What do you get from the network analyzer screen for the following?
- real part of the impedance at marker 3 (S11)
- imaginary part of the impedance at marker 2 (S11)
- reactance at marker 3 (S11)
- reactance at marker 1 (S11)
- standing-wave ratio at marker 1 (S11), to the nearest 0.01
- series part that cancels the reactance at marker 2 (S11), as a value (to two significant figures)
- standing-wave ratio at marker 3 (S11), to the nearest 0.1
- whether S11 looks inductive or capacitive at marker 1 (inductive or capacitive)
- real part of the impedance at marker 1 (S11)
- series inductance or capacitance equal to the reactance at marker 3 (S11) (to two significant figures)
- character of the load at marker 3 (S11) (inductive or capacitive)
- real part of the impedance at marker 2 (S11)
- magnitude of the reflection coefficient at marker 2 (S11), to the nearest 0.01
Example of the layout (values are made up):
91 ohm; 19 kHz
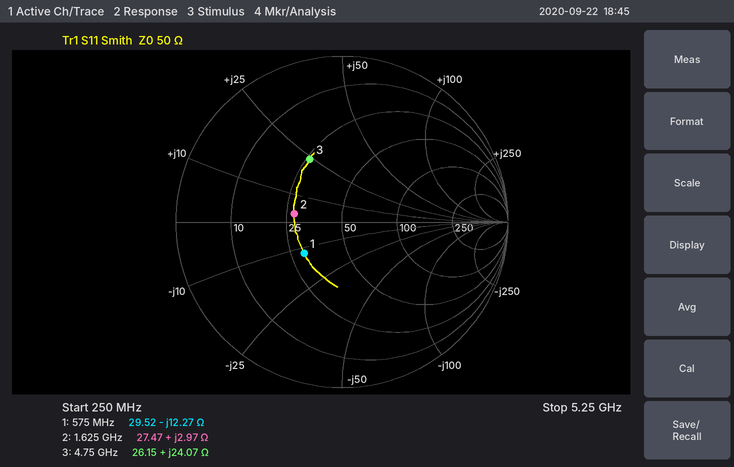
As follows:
26.15 Ω; +2.97 Ω; +24.07 Ω; -12.27 Ω; 1.84; 33 pF; 2.5; capacitive; 29.52 Ω; 810 pH; inductive; 27.47 Ω; 0.29
